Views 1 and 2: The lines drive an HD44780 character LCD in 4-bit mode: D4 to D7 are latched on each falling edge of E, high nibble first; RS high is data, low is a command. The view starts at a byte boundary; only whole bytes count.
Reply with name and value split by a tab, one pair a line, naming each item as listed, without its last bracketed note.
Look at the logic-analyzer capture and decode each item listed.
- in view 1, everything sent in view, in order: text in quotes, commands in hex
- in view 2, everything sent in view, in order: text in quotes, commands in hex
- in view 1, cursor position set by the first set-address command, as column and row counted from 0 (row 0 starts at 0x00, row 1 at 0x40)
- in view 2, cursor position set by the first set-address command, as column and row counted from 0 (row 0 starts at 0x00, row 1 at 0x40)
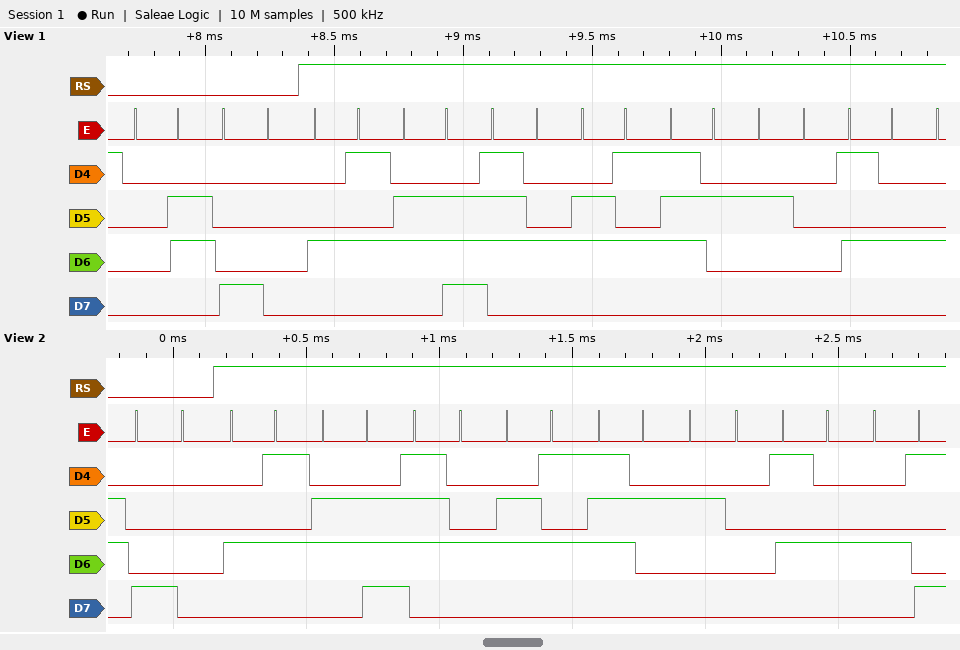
in view 1, everything sent in view, in order: text in quotes, commands in hex	0x06 0x80 "Enter T"
in view 2, everything sent in view, in order: text in quotes, commands in hex	0x80 "Enter TI"
in view 1, cursor position set by the first set-address command, as column and row counted from 0	column 0, row 0
in view 2, cursor position set by the first set-address command, as column and row counted from 0	column 0, row 0
